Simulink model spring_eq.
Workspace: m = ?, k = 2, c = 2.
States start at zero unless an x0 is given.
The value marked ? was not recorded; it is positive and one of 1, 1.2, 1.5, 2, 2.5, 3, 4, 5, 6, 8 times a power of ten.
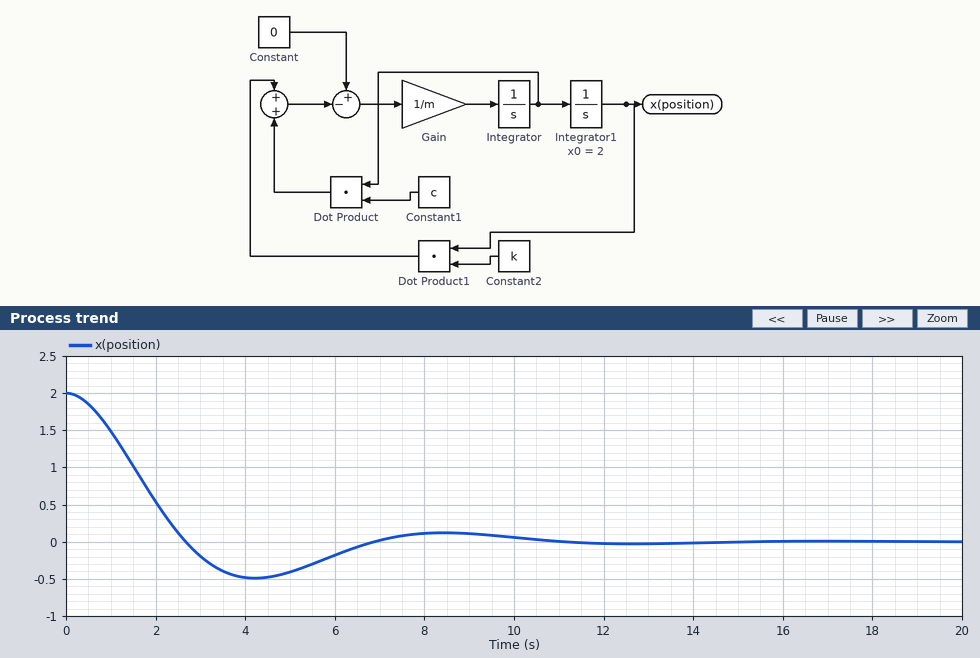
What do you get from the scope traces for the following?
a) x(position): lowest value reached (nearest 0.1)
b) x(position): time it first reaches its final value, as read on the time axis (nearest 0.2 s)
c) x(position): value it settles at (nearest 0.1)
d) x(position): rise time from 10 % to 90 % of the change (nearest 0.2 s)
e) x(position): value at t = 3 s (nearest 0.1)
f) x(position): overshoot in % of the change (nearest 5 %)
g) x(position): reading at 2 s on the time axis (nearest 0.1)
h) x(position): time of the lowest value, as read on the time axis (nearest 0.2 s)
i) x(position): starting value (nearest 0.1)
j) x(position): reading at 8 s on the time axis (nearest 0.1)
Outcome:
-0.5
2.6 s
0.0
1.8 s
-0.2
25 %
0.5
4.2 s
2.0
0.1
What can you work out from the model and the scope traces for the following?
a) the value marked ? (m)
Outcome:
3
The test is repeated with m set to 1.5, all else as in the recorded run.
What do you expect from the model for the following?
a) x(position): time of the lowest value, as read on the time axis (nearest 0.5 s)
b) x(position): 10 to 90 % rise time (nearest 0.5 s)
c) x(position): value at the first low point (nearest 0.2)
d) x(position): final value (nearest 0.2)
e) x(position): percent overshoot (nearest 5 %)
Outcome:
3.5 s
1.5 s
-0.2
0.0
10 %
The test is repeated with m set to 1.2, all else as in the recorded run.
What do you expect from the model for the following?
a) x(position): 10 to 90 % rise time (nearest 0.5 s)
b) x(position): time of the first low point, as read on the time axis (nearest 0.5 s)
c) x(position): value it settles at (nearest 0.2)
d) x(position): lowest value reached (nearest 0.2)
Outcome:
1.5 s
3.0 s
0.0
-0.2
